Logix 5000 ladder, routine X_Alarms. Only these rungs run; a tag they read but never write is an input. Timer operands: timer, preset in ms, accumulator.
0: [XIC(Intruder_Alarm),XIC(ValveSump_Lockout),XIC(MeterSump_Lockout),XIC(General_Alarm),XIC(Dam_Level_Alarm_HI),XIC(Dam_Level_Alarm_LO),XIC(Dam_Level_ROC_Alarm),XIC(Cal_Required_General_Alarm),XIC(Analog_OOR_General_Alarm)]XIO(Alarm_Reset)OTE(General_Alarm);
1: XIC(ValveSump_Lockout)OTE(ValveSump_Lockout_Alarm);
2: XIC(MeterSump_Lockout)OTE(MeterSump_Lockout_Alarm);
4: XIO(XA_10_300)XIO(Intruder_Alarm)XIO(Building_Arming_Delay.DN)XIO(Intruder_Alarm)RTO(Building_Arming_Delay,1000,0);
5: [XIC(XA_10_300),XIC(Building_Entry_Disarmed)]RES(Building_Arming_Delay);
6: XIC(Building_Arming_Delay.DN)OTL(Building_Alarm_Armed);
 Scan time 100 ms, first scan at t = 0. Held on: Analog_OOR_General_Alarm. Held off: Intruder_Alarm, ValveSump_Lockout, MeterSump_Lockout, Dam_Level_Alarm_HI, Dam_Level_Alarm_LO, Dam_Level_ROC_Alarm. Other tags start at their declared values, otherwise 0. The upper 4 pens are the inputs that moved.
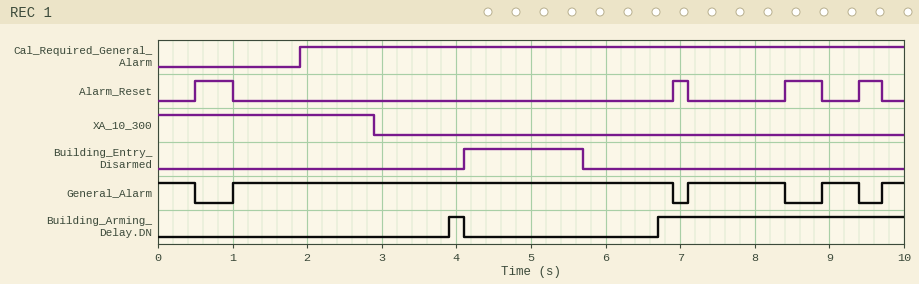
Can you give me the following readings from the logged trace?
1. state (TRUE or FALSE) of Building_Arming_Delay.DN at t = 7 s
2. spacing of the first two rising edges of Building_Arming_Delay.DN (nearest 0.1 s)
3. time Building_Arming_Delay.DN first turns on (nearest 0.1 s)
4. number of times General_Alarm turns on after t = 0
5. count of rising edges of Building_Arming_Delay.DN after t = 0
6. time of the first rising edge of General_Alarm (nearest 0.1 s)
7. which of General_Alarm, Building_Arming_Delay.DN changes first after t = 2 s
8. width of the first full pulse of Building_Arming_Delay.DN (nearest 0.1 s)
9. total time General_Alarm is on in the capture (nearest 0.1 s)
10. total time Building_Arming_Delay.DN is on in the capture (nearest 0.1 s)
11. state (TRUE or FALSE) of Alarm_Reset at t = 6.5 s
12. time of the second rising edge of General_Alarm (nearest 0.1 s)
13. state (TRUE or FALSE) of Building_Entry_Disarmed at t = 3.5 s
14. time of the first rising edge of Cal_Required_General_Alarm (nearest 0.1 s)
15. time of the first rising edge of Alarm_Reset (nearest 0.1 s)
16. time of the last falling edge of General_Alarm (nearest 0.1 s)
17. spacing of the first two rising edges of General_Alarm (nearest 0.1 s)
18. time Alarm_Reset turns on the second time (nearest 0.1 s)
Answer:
TRUE
2.8 s
3.9 s
4
2
1.0 s
Building_Arming_Delay.DN
0.2 s
8.5 s
3.5 s
FALSE
7.1 s
FALSE
1.9 s
0.5 s
9.4 s
6.1 s
6.9 s
